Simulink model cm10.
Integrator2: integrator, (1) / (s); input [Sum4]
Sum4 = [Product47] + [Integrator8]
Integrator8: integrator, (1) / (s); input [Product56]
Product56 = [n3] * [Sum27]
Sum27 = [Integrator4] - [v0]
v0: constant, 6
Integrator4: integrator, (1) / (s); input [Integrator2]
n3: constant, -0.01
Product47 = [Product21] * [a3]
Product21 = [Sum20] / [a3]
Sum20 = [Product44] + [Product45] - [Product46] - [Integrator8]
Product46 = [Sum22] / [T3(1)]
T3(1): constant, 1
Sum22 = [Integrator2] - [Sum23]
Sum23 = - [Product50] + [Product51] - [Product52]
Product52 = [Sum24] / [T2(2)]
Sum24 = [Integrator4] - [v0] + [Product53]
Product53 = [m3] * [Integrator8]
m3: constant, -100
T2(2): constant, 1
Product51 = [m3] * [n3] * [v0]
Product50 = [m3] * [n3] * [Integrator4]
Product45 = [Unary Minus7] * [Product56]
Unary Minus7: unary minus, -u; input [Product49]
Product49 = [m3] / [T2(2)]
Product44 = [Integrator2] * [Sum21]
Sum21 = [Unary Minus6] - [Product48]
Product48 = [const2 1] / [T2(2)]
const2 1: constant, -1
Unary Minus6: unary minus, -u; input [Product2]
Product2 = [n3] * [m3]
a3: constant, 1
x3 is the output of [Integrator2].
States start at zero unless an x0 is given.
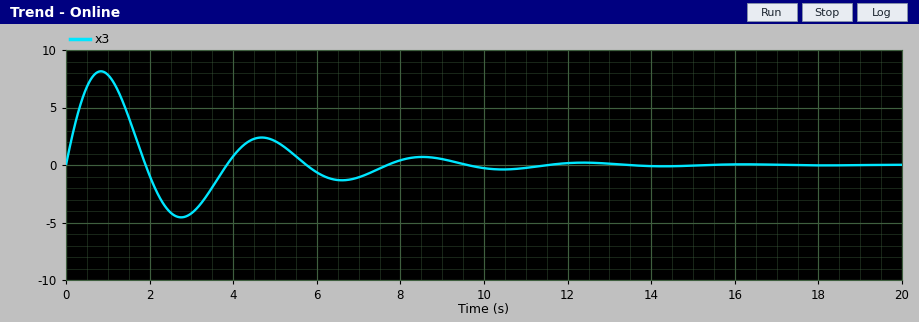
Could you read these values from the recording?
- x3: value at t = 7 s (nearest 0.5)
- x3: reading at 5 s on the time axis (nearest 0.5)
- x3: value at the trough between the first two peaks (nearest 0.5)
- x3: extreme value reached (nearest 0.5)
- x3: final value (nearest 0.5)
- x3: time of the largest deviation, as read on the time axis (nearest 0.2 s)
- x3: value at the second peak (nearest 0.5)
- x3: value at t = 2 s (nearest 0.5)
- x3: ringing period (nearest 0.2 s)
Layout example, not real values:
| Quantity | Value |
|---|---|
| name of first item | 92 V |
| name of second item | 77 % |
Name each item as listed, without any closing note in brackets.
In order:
| Quantity | Value |
|---|---|
| x3: value at t = 7 s | -1.0 |
| x3: reading at 5 s on the time axis | 2.0 |
| x3: value at the trough between the first two peaks | -4.5 |
| x3: extreme value reached | 8.0 |
| x3: final value | 0.0 |
| x3: time of the largest deviation, as read on the time axis | 0.8 s |
| x3: value at the second peak | 2.5 |
| x3: value at t = 2 s | -1.0 |
| x3: ringing period | 3.8 s |
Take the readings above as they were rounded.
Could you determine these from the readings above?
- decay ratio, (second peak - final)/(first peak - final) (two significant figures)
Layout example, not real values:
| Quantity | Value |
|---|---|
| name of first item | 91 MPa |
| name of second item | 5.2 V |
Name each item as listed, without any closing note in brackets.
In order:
| Quantity | Value |
|---|---|
| decay ratio, (second peak - final)/(first peak - final) | 0.31 |
